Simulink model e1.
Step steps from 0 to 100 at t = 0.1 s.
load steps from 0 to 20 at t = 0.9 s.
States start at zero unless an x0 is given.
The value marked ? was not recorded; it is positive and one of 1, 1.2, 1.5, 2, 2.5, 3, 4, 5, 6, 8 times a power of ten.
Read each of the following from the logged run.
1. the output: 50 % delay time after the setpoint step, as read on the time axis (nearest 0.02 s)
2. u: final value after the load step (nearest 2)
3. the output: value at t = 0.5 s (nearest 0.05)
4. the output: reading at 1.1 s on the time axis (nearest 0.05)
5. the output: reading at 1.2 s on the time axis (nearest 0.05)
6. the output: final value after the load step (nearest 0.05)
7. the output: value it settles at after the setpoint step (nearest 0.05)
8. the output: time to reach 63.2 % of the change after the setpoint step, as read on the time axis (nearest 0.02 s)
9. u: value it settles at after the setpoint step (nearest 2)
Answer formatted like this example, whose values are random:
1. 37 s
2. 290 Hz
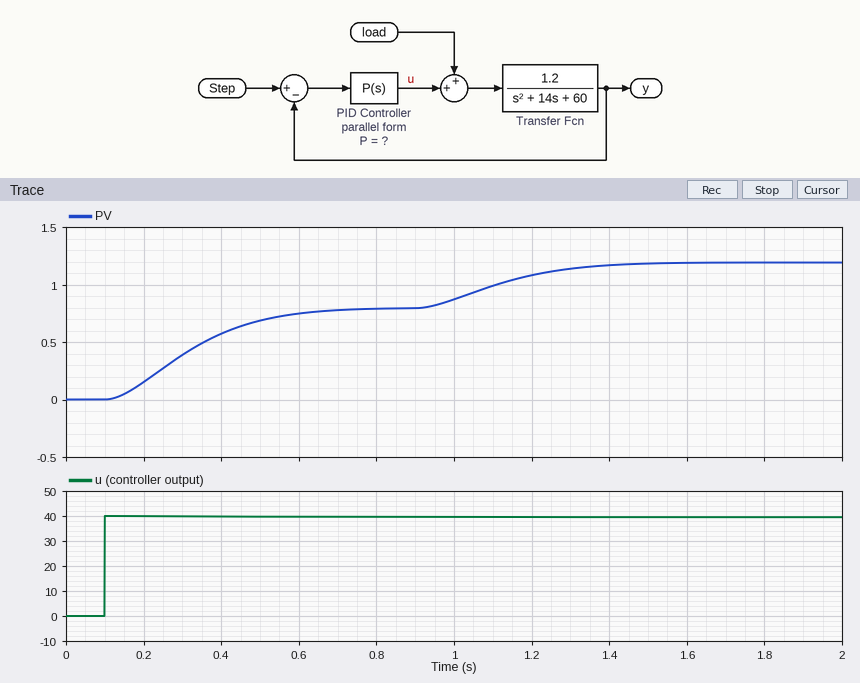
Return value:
1. 0.30 s
2. 40
3. 0.70
4. 1.00
5. 1.10
6. 1.20
7. 0.80
8. 0.36 s
9. 40
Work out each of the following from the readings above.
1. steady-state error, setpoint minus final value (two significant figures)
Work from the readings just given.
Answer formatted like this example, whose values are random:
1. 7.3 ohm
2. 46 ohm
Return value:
1. 99
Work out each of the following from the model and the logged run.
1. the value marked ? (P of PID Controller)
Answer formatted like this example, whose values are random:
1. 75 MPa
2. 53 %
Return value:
1. 0.4
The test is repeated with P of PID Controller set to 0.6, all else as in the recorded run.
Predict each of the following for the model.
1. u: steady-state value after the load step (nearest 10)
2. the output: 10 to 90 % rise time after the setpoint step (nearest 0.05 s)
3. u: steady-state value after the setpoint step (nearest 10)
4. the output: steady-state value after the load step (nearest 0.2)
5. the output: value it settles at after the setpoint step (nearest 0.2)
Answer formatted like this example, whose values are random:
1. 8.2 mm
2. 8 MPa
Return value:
1. 60
2. 0.35 s
3. 60
4. 1.6
5. 1.2
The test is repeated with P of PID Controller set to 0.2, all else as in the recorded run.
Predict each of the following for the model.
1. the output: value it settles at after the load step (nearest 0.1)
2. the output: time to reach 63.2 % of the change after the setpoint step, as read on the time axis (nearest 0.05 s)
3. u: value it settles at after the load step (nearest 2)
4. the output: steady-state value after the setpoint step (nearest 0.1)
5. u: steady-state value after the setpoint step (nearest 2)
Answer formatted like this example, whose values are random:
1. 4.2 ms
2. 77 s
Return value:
1. 0.8
2. 0.35 s
3. 20
4. 0.4
5. 20
